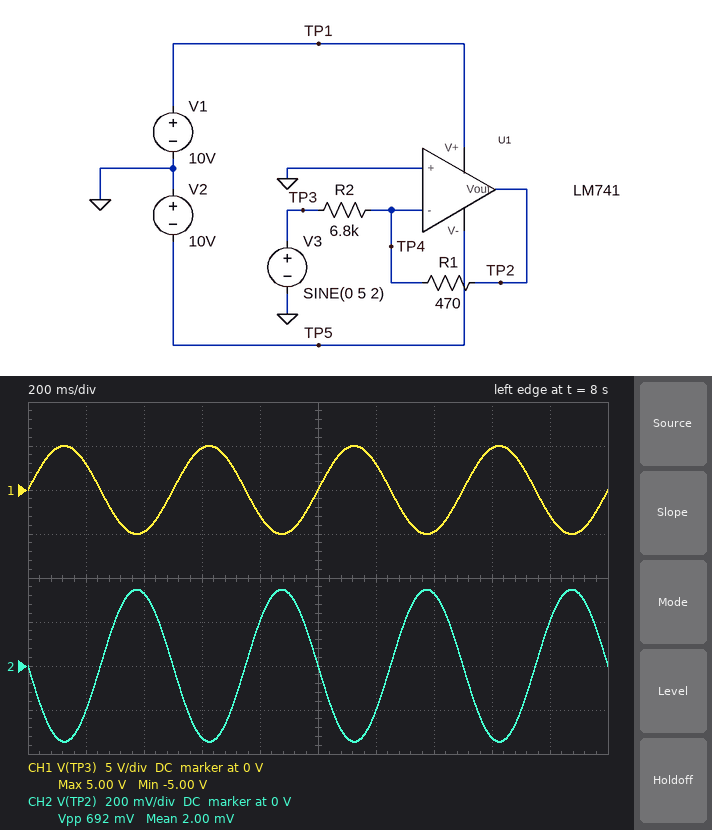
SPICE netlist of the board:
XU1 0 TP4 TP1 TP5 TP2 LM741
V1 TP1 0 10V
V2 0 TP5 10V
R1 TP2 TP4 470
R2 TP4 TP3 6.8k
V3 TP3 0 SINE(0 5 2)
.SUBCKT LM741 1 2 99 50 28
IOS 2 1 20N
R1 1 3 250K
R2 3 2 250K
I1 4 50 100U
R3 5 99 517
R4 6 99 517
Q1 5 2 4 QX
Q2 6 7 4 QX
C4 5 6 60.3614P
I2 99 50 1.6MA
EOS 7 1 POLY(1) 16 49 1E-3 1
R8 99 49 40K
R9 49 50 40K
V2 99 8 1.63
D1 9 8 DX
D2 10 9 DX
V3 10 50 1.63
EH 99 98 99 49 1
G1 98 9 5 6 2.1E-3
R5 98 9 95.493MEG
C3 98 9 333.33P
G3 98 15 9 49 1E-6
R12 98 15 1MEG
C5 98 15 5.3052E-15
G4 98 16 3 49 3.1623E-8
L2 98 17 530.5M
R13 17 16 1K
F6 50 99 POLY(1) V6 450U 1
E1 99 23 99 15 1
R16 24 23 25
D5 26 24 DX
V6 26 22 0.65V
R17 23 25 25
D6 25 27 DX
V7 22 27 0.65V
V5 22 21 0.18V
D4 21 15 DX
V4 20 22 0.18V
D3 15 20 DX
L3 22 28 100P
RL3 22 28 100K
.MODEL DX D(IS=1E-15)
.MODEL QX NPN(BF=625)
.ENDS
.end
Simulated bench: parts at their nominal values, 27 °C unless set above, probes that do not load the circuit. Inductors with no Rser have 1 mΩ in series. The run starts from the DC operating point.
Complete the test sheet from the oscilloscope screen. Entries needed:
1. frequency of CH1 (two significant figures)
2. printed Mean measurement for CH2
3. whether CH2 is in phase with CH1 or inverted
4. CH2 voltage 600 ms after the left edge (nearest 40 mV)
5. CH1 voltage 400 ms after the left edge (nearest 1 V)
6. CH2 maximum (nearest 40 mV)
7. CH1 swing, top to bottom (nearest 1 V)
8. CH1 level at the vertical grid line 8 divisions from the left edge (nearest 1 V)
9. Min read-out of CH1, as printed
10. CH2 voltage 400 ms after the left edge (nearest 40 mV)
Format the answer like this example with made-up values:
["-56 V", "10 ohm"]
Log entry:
["2.0 Hz", "2.00 mV", "inverted", "-320 mV", "-5 V", "360 mV", "10 V", "5 V", "-5.00 V", "320 mV"]
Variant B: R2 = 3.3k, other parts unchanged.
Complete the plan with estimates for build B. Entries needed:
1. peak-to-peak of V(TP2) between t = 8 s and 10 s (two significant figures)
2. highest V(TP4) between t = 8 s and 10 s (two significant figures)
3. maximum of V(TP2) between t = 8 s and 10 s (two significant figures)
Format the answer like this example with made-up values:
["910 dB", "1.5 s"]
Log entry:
["1.4 V", "1.0 mV", "710 mV"]
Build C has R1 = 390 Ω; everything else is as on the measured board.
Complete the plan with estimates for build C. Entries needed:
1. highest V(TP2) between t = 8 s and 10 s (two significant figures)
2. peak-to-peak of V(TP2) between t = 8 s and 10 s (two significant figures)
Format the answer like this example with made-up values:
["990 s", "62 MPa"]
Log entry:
["290 mV", "570 mV"]
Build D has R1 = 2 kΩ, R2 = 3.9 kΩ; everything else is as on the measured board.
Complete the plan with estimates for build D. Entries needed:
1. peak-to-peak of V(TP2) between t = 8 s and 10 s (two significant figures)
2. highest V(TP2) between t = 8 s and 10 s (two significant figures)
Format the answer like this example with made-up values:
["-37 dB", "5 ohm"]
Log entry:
["5.1 V", "2.6 V"]
